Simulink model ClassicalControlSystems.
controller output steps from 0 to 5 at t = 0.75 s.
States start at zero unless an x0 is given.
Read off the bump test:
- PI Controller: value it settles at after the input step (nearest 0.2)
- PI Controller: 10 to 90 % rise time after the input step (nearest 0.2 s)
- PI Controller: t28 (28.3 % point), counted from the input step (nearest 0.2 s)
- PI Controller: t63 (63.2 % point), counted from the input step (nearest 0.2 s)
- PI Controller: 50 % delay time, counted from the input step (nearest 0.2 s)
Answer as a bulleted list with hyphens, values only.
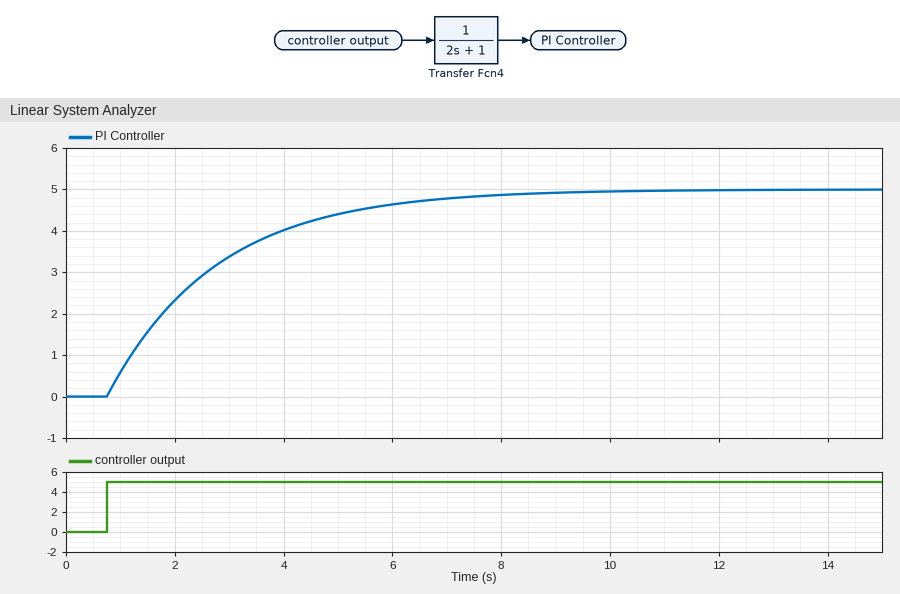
- 5.0
- 4.4 s
- 0.6 s
- 2.0 s
- 1.4 s
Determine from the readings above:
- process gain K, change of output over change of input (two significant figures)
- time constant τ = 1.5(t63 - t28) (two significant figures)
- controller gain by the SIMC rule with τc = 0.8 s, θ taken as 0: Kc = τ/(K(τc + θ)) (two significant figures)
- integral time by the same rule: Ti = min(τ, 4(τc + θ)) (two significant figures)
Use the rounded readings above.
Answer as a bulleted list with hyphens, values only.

- 1.0
- 2.1 s
- 2.6
- 2.1 s
